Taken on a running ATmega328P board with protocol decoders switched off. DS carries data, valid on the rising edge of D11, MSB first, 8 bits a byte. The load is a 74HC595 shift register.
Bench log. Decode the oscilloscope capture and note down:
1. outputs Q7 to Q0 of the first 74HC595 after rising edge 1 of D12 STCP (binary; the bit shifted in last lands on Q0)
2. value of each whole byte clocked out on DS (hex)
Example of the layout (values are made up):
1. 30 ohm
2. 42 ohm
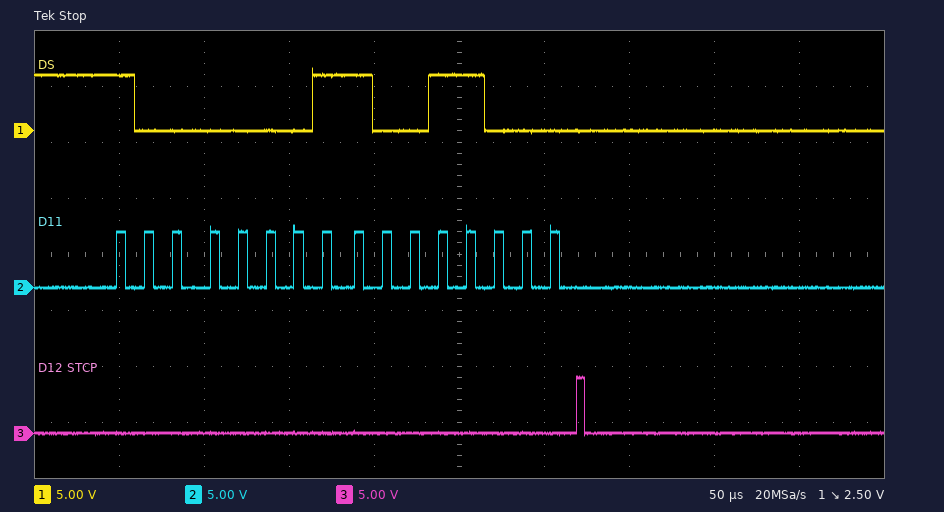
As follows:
1. 10011000
2. 81 98
